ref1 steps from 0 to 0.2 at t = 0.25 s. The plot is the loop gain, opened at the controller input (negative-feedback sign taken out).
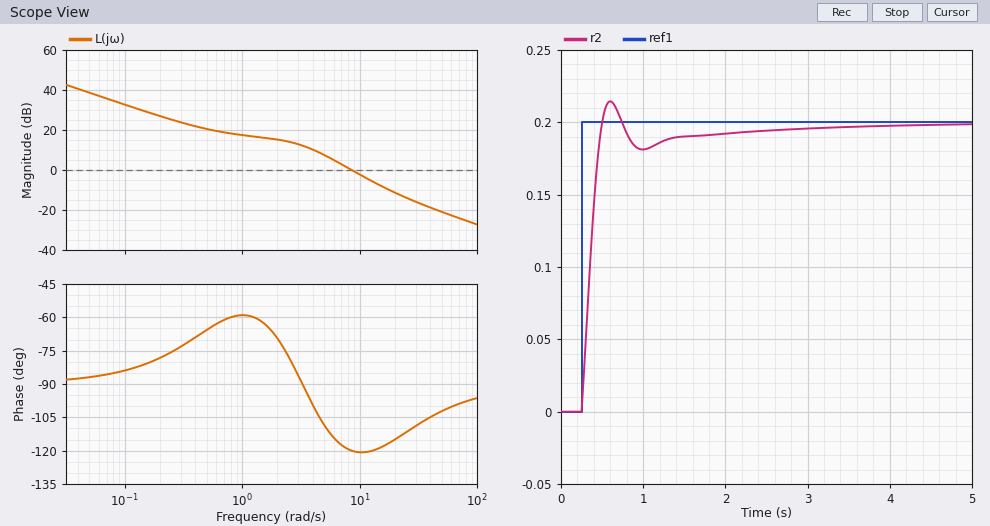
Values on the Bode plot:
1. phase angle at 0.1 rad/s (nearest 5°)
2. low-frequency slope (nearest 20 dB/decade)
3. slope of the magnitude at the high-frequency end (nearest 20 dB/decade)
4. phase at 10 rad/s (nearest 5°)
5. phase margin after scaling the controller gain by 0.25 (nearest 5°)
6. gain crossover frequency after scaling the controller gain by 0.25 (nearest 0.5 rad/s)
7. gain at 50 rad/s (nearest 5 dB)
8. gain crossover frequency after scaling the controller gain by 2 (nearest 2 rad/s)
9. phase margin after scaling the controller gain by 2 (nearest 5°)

-85°
-20 dB/decade
-20 dB/decade
-120°
90°
3.5 rad/s
-20 dB
14 rad/s
60°
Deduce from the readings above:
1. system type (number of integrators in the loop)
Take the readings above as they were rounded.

1
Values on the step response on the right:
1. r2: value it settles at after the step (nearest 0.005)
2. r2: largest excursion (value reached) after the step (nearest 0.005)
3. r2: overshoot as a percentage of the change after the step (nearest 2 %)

0.200
0.215
8 %
